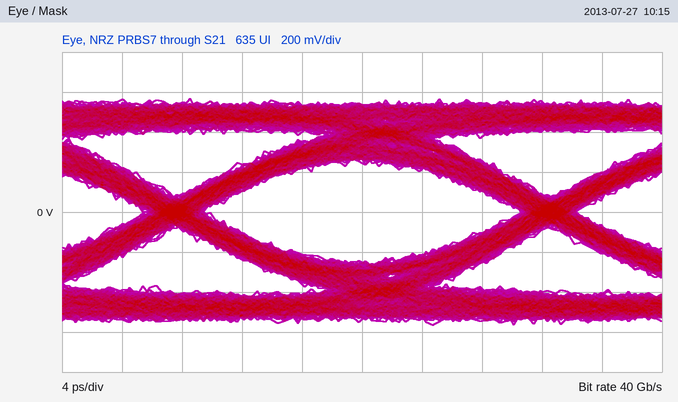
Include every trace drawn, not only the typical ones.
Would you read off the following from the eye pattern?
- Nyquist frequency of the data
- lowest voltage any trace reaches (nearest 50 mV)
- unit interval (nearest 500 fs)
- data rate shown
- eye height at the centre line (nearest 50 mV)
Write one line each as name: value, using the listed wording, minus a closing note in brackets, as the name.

Nyquist frequency of the data: 20 GHz
lowest voltage any trace reaches: -550 mV
unit interval: 25.0 ps
data rate shown: 40 Gb/s
eye height at the centre line: 500 mV
